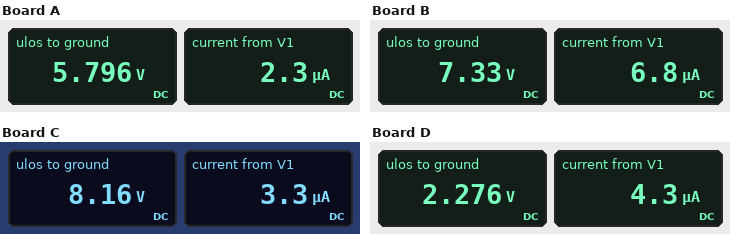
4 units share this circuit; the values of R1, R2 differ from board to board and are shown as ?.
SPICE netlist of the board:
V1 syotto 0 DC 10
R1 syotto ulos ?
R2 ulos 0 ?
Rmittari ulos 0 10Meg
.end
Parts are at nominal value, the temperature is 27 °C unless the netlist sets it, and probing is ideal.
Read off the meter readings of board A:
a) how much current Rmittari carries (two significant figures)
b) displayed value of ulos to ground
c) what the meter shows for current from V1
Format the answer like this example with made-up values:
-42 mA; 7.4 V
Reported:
580 nA; 5.796 V; 2.3 µA
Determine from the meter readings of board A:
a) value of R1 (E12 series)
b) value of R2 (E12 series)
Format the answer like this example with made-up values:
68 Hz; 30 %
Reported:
1.8 MΩ; 3.3 MΩ
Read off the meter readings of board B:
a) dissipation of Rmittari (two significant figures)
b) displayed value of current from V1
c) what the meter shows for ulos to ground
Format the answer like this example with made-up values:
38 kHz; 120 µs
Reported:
5.4 µW; 6.8 µA; 7.33 V
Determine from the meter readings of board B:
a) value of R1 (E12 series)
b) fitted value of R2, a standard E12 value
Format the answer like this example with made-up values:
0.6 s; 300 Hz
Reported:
390 kΩ; 1.2 MΩ
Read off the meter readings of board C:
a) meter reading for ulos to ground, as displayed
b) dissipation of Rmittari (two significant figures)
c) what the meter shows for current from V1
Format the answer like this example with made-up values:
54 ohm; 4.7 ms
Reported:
8.16 V; 6.7 µW; 3.3 µA
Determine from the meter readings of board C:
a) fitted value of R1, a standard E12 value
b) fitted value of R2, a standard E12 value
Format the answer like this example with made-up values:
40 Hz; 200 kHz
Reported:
560 kΩ; 3.3 MΩ
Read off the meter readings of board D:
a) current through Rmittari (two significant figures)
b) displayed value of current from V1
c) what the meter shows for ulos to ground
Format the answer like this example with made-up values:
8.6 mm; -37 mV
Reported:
230 nA; 4.3 µA; 2.276 V
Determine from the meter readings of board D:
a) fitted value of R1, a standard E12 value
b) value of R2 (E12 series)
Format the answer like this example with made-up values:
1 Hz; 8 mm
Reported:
1.8 MΩ; 560 kΩ
